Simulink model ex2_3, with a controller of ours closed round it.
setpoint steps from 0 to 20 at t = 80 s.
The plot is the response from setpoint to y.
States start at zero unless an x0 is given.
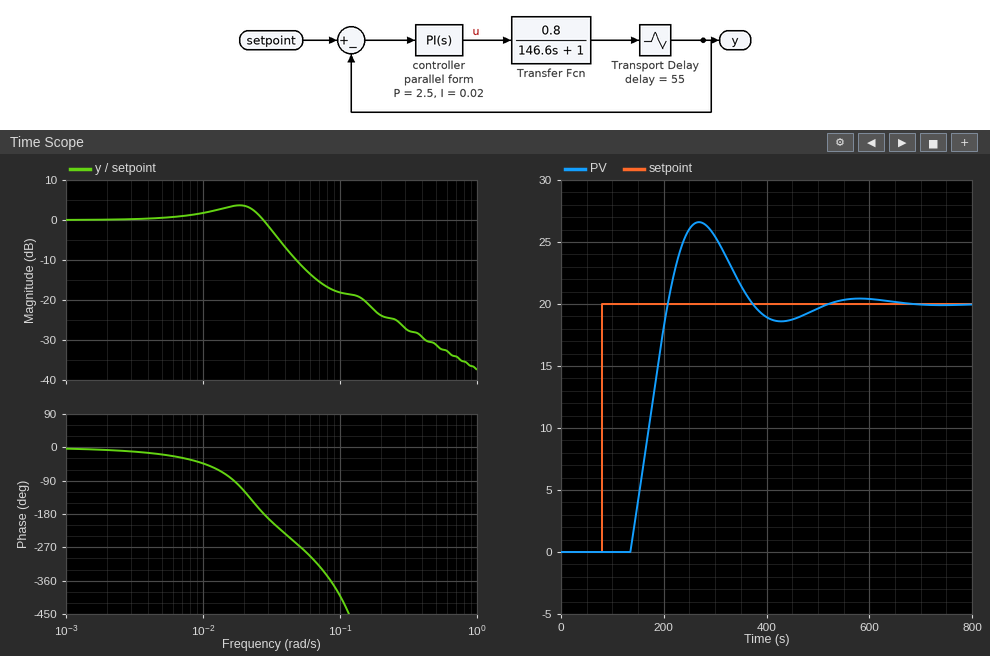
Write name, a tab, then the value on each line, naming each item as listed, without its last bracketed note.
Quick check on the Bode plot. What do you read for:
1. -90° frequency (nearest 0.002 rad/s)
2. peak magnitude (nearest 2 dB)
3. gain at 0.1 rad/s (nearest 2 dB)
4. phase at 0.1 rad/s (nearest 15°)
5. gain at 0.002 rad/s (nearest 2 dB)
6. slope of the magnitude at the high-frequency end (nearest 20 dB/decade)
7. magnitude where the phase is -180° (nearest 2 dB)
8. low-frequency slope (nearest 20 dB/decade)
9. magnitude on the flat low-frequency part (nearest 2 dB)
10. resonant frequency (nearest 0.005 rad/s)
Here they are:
-90° frequency	0.016 rad/s
peak magnitude	4 dB
gain at 0.1 rad/s	-18 dB
phase at 0.1 rad/s	-405°
gain at 0.002 rad/s	0 dB
slope of the magnitude at the high-frequency end	-20 dB/decade
magnitude where the phase is -180°	0 dB
low-frequency slope	0 dB/decade
magnitude on the flat low-frequency part	0 dB
resonant frequency	0.020 rad/s
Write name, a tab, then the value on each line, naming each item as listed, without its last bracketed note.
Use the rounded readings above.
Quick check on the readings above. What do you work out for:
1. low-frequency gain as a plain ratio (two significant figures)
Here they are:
low-frequency gain as a plain ratio	1.0
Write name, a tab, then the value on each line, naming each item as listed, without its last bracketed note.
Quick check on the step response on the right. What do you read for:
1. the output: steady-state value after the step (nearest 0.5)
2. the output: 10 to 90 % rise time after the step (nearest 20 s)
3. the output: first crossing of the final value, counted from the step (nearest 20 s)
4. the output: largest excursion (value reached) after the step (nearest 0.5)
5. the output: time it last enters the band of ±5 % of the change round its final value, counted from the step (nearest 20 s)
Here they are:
the output: steady-state value after the step	20.0
the output: 10 to 90 % rise time after the step	60 s
the output: first crossing of the final value, counted from the step	120 s
the output: largest excursion (value reached) after the step	26.5
the output: time it last enters the band of ±5 % of the change round its final value, counted from the step	380 s
